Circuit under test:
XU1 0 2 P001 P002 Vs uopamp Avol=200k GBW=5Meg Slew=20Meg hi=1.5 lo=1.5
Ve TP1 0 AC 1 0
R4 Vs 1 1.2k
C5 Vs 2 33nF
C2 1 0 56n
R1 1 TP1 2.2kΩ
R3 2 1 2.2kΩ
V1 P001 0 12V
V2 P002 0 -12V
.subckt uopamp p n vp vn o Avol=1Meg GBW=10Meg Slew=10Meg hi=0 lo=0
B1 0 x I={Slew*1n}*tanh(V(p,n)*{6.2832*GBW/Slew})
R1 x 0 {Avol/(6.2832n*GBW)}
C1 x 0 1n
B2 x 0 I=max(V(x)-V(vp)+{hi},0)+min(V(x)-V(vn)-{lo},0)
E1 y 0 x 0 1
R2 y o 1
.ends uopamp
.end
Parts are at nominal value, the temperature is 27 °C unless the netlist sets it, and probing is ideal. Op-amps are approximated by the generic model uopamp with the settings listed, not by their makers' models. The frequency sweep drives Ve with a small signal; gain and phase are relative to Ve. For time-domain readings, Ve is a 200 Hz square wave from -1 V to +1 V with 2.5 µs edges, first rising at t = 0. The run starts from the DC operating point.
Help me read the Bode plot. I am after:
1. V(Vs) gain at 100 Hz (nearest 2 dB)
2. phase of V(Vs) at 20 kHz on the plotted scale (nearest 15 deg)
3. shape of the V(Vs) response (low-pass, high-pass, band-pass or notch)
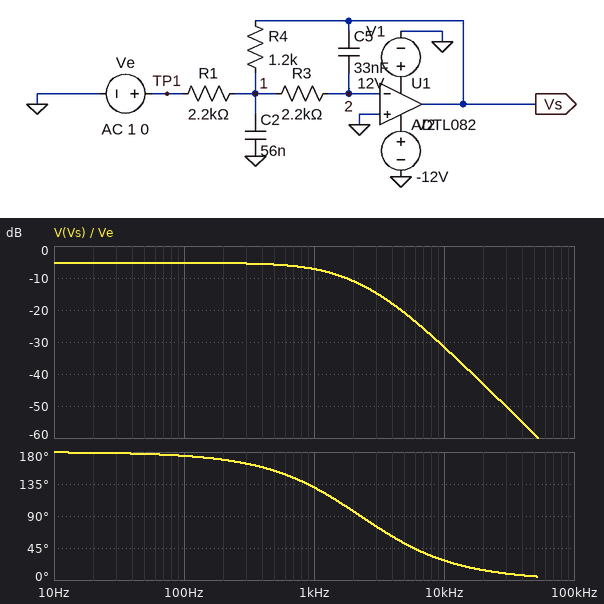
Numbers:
-6 dB
15 deg
low-pass
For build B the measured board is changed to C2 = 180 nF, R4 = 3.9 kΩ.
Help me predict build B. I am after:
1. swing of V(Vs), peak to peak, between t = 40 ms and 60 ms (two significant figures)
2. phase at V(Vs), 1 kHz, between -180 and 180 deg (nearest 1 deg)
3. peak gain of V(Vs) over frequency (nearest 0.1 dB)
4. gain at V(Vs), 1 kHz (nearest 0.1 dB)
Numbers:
3.8 V
64 deg
5.0 dB
-2.3 dB
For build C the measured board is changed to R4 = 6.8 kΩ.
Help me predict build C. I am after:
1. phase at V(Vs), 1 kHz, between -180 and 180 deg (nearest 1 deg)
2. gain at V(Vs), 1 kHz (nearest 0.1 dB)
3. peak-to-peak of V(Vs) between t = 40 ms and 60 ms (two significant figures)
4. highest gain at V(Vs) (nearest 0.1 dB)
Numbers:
88 deg
-0.5 dB
6.1 V
9.8 dB
